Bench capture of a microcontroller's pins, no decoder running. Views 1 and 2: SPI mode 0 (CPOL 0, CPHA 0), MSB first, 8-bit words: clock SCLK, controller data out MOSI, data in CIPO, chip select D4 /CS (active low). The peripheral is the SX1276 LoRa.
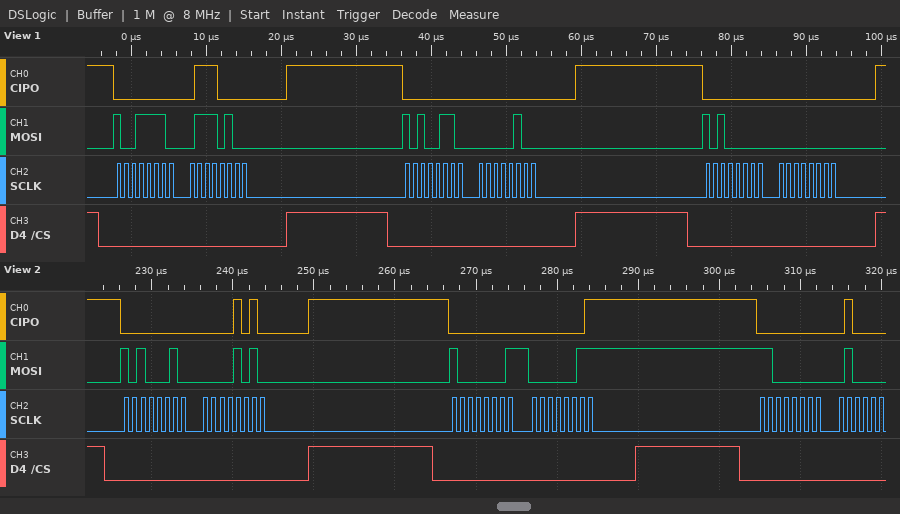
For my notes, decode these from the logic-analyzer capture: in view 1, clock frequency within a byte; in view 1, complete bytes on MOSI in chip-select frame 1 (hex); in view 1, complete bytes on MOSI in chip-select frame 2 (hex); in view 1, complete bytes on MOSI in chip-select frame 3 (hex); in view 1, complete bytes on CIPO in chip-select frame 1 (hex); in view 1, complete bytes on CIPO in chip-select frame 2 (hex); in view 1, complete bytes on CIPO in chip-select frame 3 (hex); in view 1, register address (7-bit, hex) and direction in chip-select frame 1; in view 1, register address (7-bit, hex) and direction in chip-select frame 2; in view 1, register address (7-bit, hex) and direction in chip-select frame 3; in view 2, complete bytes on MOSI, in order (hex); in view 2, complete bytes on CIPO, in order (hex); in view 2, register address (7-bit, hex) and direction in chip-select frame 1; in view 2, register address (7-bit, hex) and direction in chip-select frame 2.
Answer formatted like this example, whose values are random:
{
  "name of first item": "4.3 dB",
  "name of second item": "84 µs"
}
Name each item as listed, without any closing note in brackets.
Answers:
{
  "in view 1, clock frequency within a byte": "1 MHz",
  "in view 1, complete bytes on MOSI in chip-select frame 1": "9E 74",
  "in view 1, complete bytes on MOSI in chip-select frame 2": "A6 04",
  "in view 1, complete bytes on MOSI in chip-select frame 3": "A0 00",
  "in view 1, complete bytes on CIPO in chip-select frame 1": "00 70",
  "in view 1, complete bytes on CIPO in chip-select frame 2": "00 00",
  "in view 1, complete bytes on CIPO in chip-select frame 3": "00 00",
  "in view 1, register address (7-bit, hex) and direction in chip-select frame 1": "0x1E write",
  "in view 1, register address (7-bit, hex) and direction in chip-select frame 2": "0x26 write",
  "in view 1, register address (7-bit, hex) and direction in chip-select frame 3": "0x20 write",
  "in view 2, complete bytes on MOSI, in order": "0xA2 0x0A 0x81 0x03 0xC0",
  "in view 2, complete bytes on CIPO, in order": "0x00 0x0A 0x00 0x01 0x00",
  "in view 2, register address (7-bit, hex) and direction in chip-select frame 1": "0x22 write",
  "in view 2, register address (7-bit, hex) and direction in chip-select frame 2": "0x01 write"
}
